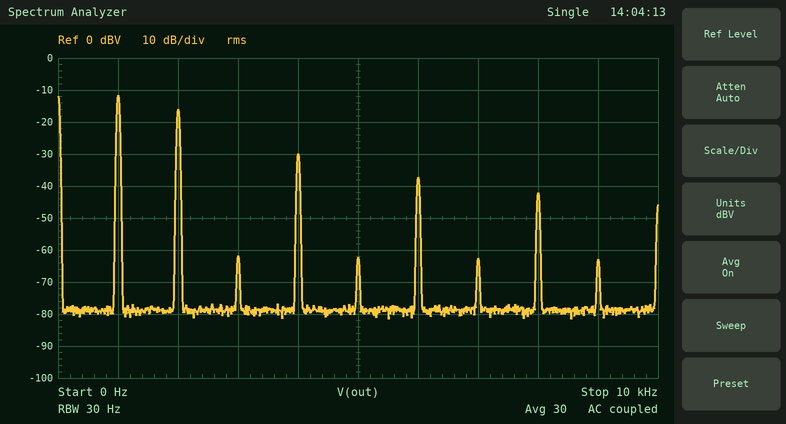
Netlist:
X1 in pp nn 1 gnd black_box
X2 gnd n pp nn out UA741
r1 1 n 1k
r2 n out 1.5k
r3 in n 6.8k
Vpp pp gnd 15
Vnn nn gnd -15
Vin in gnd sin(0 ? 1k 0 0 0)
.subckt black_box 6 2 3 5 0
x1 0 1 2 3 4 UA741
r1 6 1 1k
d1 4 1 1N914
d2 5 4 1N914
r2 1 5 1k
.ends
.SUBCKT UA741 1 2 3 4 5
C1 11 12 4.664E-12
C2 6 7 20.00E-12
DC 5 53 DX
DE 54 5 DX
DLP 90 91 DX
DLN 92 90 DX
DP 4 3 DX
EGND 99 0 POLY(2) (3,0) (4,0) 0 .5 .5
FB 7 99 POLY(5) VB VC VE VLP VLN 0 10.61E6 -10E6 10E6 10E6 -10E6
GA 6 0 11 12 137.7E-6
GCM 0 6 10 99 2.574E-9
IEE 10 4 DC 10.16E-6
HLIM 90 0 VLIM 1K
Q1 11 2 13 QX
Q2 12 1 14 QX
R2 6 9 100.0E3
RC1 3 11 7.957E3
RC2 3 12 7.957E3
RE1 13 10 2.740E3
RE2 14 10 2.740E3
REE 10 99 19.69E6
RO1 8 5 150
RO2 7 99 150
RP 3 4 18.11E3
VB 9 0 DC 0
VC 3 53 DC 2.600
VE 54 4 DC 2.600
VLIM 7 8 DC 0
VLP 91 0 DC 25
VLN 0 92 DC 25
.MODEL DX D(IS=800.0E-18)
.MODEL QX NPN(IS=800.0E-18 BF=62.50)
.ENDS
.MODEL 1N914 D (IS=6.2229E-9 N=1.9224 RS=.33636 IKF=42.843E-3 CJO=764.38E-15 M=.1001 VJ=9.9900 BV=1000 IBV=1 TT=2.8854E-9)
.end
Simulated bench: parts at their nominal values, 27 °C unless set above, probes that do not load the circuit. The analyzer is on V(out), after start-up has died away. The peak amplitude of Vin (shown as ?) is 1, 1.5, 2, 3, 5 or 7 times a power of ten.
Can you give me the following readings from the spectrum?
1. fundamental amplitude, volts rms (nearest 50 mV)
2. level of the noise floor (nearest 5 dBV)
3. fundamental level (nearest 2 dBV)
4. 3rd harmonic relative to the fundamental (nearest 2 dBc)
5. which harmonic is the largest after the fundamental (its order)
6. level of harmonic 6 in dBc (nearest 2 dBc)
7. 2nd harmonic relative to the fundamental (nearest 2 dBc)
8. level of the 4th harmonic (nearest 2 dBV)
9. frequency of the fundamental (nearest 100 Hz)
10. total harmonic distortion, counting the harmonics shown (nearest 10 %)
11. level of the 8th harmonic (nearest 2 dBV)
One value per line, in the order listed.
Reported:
250 mV
-80 dBV
-12 dBV
-50 dBc
2
-26 dBc
-4 dBc
-30 dBV
1.0 kHz
60 %
-42 dBV
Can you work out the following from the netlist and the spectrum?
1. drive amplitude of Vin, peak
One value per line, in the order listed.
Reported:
700 mV
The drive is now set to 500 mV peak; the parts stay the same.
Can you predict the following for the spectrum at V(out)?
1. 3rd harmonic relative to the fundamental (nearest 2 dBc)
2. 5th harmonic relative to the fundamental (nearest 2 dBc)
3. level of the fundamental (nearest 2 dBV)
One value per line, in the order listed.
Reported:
-48 dBc
-48 dBc
-14 dBV
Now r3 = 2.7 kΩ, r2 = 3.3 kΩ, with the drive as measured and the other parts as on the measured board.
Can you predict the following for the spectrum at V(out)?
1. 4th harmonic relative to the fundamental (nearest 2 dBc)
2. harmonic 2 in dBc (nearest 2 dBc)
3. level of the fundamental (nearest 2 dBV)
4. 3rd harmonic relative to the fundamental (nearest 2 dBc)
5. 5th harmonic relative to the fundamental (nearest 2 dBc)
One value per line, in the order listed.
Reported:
-10 dBc
4 dBc
-14 dBV
-42 dBc
-42 dBc
